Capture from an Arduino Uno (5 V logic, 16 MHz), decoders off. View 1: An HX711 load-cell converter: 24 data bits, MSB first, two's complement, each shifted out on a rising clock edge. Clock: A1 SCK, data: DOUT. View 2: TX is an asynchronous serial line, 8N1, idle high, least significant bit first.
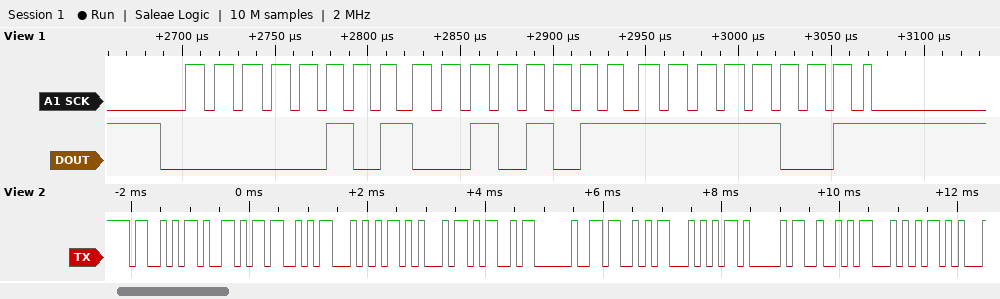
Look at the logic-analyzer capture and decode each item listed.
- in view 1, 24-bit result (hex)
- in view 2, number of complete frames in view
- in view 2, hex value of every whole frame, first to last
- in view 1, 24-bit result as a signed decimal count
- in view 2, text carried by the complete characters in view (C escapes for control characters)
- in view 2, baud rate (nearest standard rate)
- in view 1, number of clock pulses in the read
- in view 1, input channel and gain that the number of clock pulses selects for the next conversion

0x052BF9
12
0x53 0x59 0x53 0x54 0x45 0x4D 0x20 0x53 0x54 0x41 0x52 0x54
338937
"SYSTEM START"
9600 baud
25
channel A, gain 128
